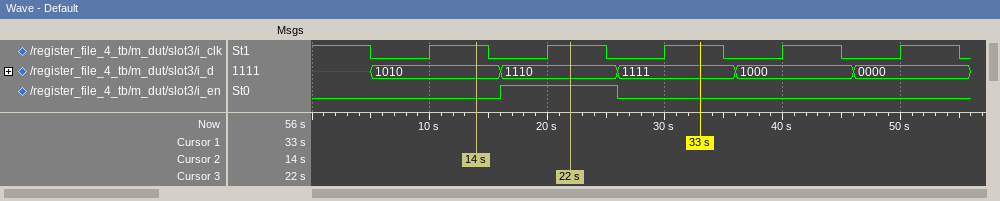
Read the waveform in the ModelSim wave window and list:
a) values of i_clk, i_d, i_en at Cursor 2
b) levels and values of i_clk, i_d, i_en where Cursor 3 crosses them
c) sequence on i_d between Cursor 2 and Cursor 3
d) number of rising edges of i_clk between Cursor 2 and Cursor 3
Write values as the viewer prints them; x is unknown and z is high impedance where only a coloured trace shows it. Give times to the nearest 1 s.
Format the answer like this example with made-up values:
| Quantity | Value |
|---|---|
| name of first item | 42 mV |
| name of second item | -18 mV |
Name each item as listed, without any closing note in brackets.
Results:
| Quantity | Value |
|---|---|
| values of i_clk, i_d, i_en at Cursor 2 | i_clk=1, i_d=1010, i_en=0 |
| levels and values of i_clk, i_d, i_en where Cursor 3 crosses them | i_clk=1, i_d=1110, i_en=1 |
| sequence on i_d between Cursor 2 and Cursor 3 | 1010, 1110 |
| number of rising edges of i_clk between Cursor 2 and Cursor 3 | 1 |
